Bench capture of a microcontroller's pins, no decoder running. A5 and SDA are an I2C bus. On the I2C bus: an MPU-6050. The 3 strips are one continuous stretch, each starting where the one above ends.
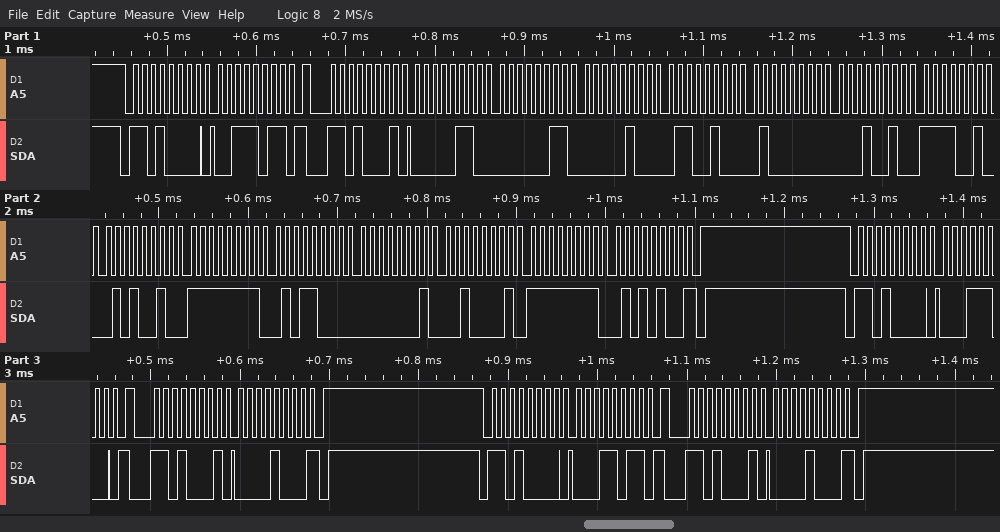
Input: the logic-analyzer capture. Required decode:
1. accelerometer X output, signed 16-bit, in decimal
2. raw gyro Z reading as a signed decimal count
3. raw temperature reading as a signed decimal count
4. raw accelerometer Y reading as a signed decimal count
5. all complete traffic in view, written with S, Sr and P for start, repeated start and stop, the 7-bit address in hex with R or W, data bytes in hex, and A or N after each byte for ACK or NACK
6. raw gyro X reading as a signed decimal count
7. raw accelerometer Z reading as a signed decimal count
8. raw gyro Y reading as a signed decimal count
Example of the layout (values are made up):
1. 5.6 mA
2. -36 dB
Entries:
1. 1539
2. -172
3. -3502
4. 1124
5. S 68W A 3B A Sr 68R A 06 A 03 A 04 A 64 A 40 A 12 A F2 A 52 A FF A 58 A 01 A 21 A FF A 54 N P S 68W A 1C A Sr 68R A 08 N P S 68W A 1B A Sr 68R A 08 N P
6. -168
7. 16402
8. 289
